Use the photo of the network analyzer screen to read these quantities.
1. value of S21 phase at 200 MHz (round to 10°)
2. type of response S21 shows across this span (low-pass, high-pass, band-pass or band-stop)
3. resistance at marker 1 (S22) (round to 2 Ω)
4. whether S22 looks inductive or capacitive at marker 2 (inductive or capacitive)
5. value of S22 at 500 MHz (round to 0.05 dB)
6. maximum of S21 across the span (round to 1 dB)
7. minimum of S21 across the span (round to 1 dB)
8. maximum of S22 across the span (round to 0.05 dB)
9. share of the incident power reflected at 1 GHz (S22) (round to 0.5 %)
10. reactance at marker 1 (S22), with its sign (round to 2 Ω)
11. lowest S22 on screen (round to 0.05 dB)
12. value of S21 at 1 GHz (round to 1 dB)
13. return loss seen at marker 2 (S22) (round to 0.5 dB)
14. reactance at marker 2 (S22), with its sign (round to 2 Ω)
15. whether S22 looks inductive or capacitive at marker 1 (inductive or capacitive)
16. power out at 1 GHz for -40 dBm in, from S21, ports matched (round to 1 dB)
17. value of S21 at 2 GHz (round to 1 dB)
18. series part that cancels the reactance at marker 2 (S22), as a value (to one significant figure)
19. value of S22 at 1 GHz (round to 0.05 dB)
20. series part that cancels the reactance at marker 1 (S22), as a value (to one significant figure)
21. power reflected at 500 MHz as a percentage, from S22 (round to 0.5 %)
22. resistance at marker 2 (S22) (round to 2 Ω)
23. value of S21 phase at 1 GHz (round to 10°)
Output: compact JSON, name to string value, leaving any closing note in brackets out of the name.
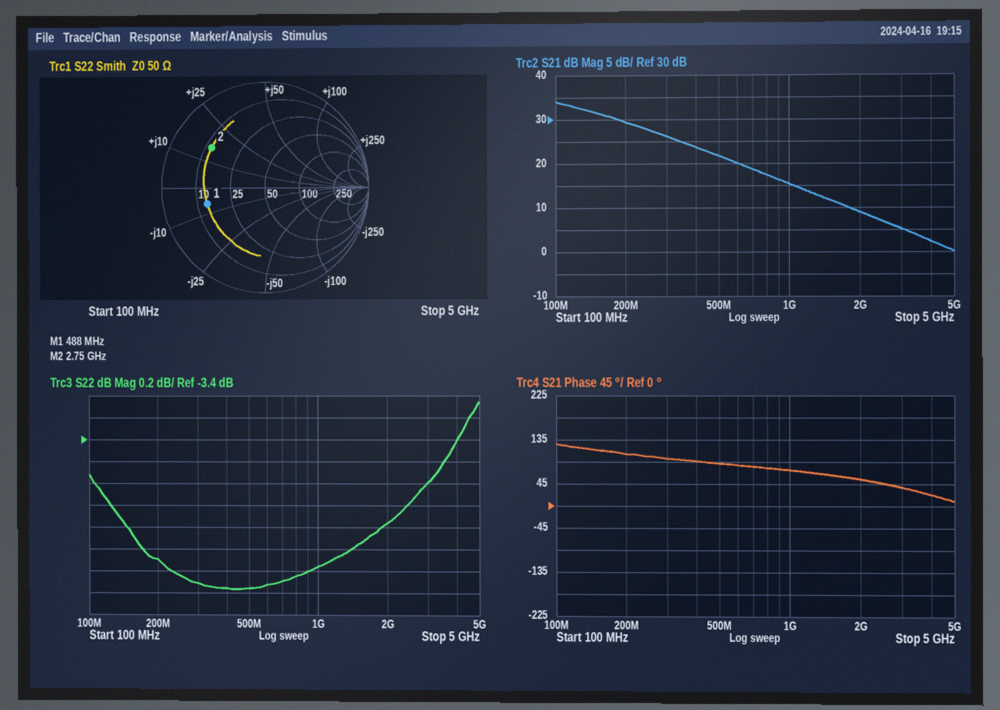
{"value of S21 phase at 200 MHz": "110°", "type of response S21 shows across this span": "low-pass", "resistance at marker 1 (S22)": "14 Ω", "whether S22 looks inductive or capacitive at marker 2": "inductive", "value of S22 at 500 MHz": "-4.75 dB", "maximum of S21 across the span": "34 dB", "minimum of S21 across the span": "0 dB", "maximum of S22 across the span": "-3.05 dB", "share of the incident power reflected at 1 GHz (S22)": "35.0 %", "reactance at marker 1 (S22), with its sign": "-6 Ω", "lowest S22 on screen": "-4.75 dB", "value of S21 at 1 GHz": "15 dB", "return loss seen at marker 2 (S22)": "4.0 dB", "reactance at marker 2 (S22), with its sign": "+16 Ω", "whether S22 looks inductive or capacitive at marker 1": "capacitive", "power out at 1 GHz for -40 dBm in, from S21, ports matched": "-25 dBm", "value of S21 at 2 GHz": "9 dB", "series part that cancels the reactance at marker 2 (S22), as a value": "4 pF", "value of S22 at 1 GHz": "-4.55 dB", "series part that cancels the reactance at marker 1 (S22), as a value": "2 nH", "power reflected at 500 MHz as a percentage, from S22": "33.5 %", "resistance at marker 2 (S22)": "12 Ω", "value of S21 phase at 1 GHz": "70°"}
